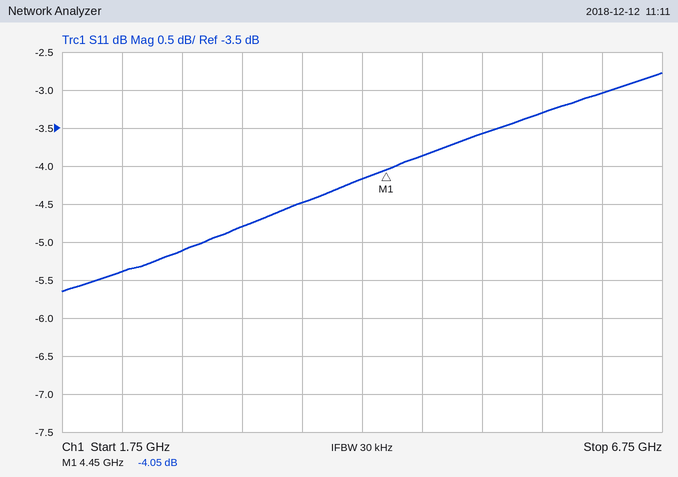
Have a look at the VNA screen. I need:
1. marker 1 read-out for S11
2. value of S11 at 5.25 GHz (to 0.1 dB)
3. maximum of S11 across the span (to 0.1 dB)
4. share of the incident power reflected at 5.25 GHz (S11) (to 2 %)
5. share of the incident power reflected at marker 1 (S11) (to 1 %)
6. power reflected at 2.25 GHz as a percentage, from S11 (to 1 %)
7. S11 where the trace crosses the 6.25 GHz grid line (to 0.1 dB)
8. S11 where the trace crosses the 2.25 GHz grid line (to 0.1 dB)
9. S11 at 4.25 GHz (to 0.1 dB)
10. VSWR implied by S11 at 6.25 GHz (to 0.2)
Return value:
-4.05 dB
-3.6 dB
-2.8 dB
44 %
39 %
29 %
-3.0 dB
-5.4 dB
-4.2 dB
5.8
